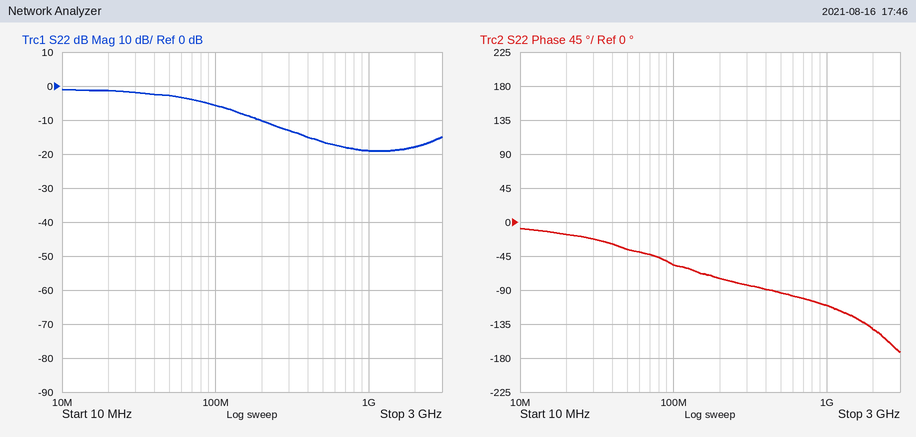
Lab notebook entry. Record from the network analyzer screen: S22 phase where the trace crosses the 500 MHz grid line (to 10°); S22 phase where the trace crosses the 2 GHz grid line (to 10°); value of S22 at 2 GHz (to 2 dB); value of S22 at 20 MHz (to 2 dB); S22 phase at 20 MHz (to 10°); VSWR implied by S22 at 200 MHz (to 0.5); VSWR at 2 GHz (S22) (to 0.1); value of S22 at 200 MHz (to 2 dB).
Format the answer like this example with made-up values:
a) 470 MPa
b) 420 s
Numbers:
a) -90°
b) -140°
c) -18 dB
d) -2 dB
e) -20°
f) 2.0
g) 1.3
h) -10 dB
